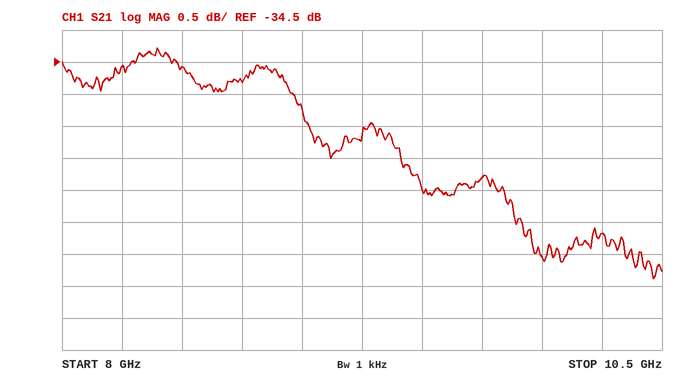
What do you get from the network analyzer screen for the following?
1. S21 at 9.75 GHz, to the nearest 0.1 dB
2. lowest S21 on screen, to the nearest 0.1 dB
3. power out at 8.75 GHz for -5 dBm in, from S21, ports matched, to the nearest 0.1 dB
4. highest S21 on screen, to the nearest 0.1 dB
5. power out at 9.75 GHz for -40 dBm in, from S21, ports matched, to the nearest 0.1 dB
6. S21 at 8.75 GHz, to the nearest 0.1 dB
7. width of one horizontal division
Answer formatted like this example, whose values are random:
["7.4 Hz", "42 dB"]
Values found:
["-36.3 dB", "-37.9 dB", "-39.8 dBm", "-34.3 dB", "-76.3 dBm", "-34.8 dB", "250 MHz"]
